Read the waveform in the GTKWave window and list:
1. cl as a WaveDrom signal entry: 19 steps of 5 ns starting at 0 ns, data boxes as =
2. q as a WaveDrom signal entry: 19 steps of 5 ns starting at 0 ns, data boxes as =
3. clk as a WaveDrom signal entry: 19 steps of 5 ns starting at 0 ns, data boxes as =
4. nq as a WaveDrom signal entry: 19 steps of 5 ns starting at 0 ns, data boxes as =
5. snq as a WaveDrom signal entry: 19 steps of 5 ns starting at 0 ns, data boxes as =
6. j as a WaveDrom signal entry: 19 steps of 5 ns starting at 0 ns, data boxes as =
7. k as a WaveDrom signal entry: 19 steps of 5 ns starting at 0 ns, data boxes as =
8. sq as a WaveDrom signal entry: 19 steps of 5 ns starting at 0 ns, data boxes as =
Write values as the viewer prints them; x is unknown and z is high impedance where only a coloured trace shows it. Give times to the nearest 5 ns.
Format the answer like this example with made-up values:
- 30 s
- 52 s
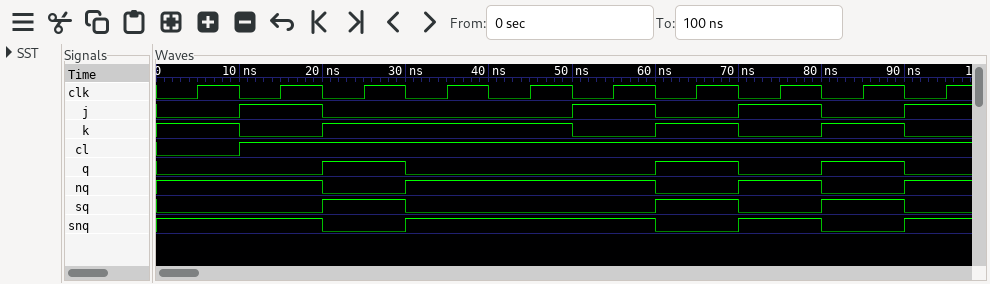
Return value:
- {name: 'cl', wave: '0.1................'}
- {name: 'q', wave: '0...1.0.....1.0.1.0'}
- {name: 'clk', wave: '0101010101010101010'}
- {name: 'nq', wave: '1...0.1.....0.1.0.1'}
- {name: 'snq', wave: '1...0.1.....0.1.0.1'}
- {name: 'j', wave: '0.1.0.....1.0.1.0.1'}
- {name: 'k', wave: '1.0.1.....0.1.0.1.0'}
- {name: 'sq', wave: '0...1.0.....1.0.1.0'}
